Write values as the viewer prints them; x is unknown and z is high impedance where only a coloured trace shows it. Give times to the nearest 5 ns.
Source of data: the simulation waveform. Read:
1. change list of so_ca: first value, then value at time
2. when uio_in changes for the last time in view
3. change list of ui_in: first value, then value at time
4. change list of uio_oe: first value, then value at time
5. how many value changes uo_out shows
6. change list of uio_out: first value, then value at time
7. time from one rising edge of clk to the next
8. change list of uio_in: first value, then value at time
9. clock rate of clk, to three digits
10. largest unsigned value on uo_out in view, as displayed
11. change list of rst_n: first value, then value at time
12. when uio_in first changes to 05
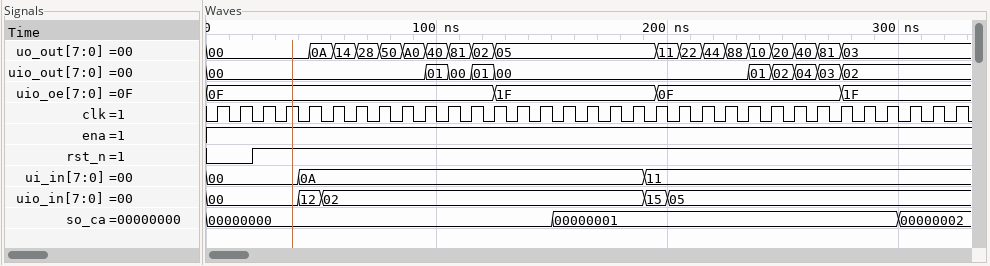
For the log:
00000000, 00000001 at 150 ns, 00000002 at 300 ns
200 ns
00, 0A at 40 ns, 11 at 190 ns
0F, 1F at 125 ns, 0F at 195 ns, 1F at 275 ns
18
00, 01 at 95 ns, 00 at 105 ns, 01 at 115 ns, 00 at 125 ns, 01 at 235 ns, 02 at 245 ns, 04 at 255 ns, 03 at 265 ns, 02 at 275 ns
10 ns
00, 12 at 40 ns, 02 at 50 ns, 15 at 190 ns, 05 at 200 ns
100 MHz
A0
0, 1 at 20 ns
200 ns
